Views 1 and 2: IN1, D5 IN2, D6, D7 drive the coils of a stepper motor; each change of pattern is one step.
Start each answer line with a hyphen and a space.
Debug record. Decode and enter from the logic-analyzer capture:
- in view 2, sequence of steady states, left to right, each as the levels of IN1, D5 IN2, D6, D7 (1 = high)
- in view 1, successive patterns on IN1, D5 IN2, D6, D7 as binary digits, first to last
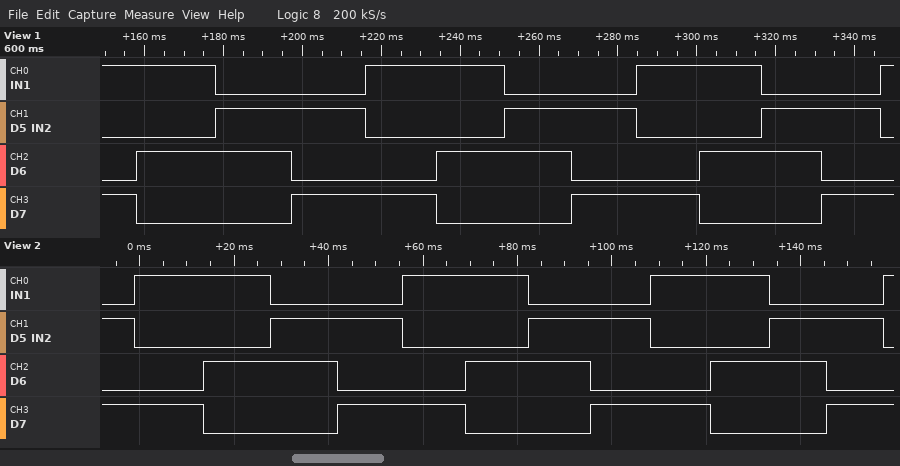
- 0101 1001 1010 0110 0101 1001 1010 0110 0101 1001 1010 0110 0101 1001
- 1001 1010 0110 0101 1001 1010 0110 0101 1001 1010 0110 0101 1001
